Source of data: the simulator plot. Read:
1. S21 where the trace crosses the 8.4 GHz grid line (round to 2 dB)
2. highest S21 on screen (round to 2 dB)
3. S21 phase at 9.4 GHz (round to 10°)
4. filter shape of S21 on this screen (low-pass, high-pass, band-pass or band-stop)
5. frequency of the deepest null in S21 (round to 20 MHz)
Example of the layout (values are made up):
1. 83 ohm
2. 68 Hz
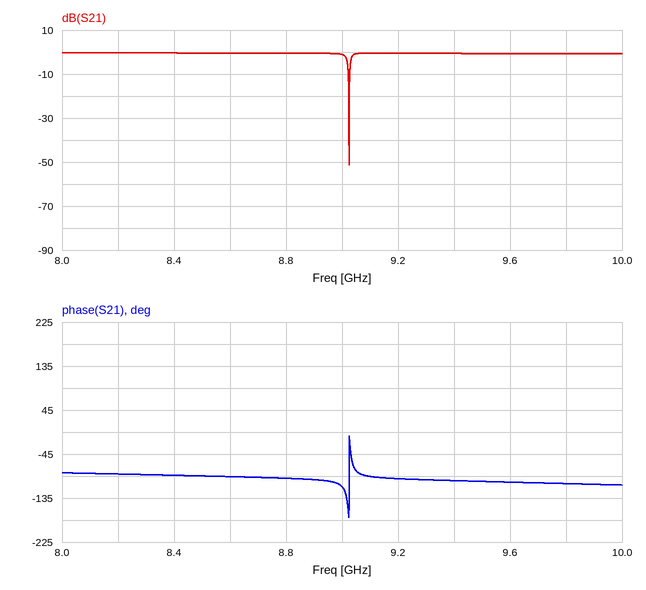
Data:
1. 0 dB
2. 0 dB
3. -100°
4. band-stop
5. 9.02 GHz
